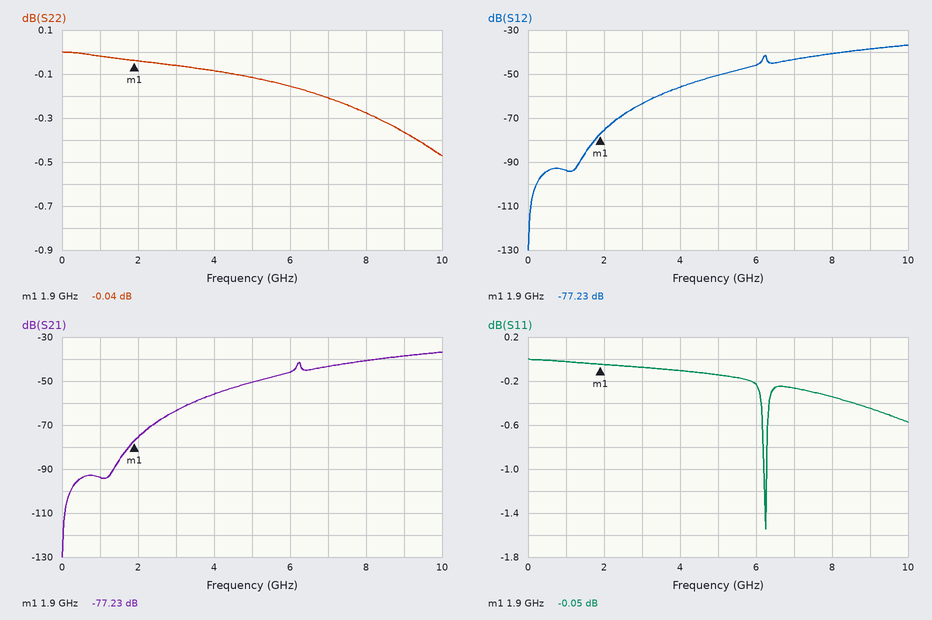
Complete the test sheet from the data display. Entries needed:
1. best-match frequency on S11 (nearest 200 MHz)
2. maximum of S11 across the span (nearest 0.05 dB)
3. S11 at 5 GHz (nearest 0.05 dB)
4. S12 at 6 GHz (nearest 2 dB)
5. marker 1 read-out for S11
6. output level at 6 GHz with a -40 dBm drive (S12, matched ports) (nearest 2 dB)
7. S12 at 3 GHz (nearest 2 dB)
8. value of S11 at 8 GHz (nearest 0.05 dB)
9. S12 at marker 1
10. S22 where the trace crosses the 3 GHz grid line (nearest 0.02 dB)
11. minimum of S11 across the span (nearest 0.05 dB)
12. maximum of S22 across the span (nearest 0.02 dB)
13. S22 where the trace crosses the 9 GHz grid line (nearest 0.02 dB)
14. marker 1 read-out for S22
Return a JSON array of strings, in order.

["6.2 GHz", "0.00 dB", "-0.15 dB", "-46 dB", "-0.05 dB", "-86 dBm", "-64 dB", "-0.35 dB", "-77.23 dB", "-0.06 dB", "-1.55 dB", "0.00 dB", "-0.36 dB", "-0.04 dB"]
